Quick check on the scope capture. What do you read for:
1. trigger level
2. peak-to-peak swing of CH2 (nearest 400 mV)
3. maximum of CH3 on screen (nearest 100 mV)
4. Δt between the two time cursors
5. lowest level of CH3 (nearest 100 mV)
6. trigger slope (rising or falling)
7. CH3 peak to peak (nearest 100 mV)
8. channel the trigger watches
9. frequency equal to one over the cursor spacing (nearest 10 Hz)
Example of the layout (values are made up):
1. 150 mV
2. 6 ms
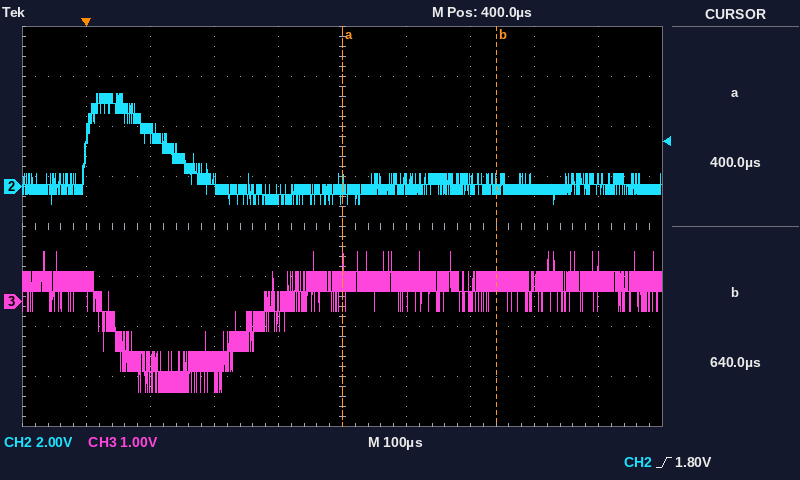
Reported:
1. 1.80 V
2. 4.4 V
3. 1.0 V
4. 240 µs
5. -1.8 V
6. rising
7. 2.8 V
8. CH2
9. 4.17 kHz
